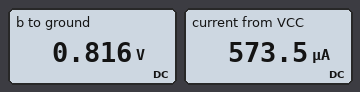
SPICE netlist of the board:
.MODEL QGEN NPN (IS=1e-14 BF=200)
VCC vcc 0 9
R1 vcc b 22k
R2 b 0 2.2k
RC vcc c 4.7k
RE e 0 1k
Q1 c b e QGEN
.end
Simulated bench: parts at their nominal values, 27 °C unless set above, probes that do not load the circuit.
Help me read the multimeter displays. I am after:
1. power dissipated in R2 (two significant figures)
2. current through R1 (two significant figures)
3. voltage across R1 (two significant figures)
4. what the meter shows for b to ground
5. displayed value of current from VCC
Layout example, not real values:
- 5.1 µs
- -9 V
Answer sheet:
- 300 µW
- 370 µA
- 8.2 V
- 0.816 V
- 573.5 µA
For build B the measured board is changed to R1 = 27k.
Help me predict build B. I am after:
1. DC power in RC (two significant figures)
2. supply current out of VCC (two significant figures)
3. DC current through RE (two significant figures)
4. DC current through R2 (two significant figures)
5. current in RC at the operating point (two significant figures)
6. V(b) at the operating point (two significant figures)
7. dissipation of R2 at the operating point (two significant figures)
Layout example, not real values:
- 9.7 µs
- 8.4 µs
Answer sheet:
- 34 µW
- 390 µA
- 86 µA
- 310 µA
- 85 µA
- 680 mV
- 210 µW
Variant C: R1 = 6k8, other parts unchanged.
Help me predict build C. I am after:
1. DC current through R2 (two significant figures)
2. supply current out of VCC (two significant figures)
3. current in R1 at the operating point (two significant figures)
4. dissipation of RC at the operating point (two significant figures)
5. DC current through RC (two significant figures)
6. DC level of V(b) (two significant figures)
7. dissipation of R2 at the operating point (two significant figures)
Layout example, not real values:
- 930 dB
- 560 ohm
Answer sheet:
- 990 µA
- 2.5 mA
- 1.0 mA
- 11 mW
- 1.5 mA
- 2.2 V
- 2.2 mW
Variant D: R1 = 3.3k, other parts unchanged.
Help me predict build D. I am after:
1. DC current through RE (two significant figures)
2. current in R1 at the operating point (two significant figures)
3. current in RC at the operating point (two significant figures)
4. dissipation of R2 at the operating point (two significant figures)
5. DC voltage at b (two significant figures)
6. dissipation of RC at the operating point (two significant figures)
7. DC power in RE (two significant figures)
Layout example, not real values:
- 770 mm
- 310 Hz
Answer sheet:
- 2.1 mA
- 1.9 mA
- 1.5 mA
- 3.5 mW
- 2.8 V
- 10 mW
- 4.4 mW
